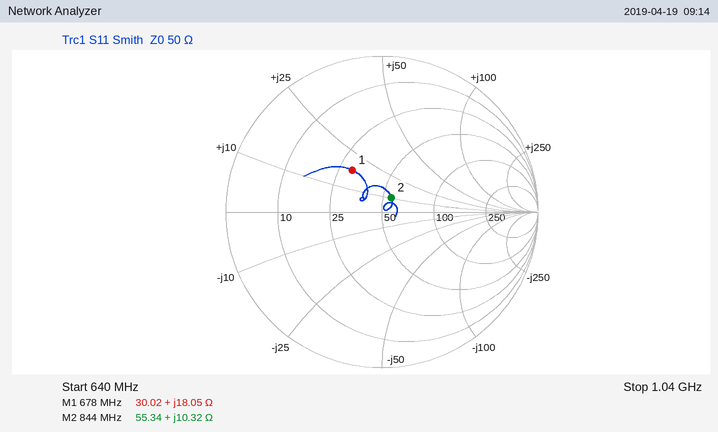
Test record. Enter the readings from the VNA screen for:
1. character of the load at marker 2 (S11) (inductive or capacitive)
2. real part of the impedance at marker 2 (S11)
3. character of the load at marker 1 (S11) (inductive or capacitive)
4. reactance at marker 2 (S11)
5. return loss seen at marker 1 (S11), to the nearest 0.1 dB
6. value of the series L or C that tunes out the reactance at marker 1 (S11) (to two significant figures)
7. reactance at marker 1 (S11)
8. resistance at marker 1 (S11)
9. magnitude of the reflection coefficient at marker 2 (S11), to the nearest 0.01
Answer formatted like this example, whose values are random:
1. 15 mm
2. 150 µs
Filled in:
1. inductive
2. 55.34 Ω
3. inductive
4. +10.32 Ω
5. 9.7 dB
6. 13 pF
7. +18.05 Ω
8. 30.02 Ω
9. 0.11
